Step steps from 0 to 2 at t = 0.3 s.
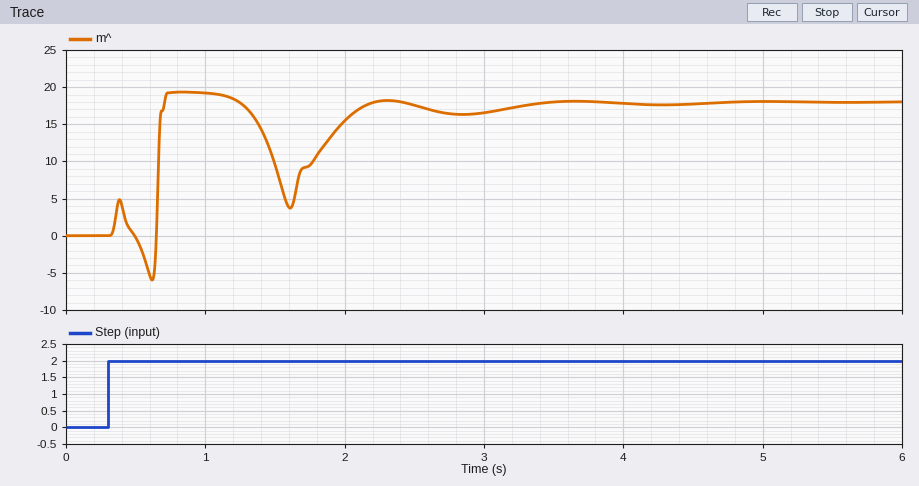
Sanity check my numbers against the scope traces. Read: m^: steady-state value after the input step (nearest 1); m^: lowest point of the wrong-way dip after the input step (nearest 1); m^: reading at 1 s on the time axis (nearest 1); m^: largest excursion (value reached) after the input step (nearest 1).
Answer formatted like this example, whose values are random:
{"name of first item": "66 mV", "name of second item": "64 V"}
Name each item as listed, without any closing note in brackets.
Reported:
{"m^: steady-state value after the input step": "18", "m^: lowest point of the wrong-way dip after the input step": "-6", "m^: reading at 1 s on the time axis": "19", "m^: largest excursion (value reached) after the input step": "19"}
